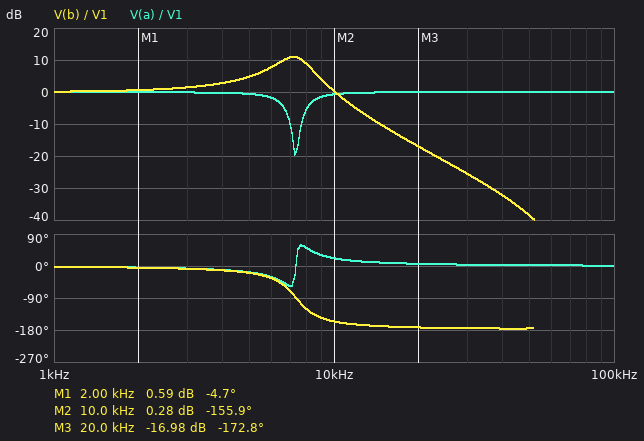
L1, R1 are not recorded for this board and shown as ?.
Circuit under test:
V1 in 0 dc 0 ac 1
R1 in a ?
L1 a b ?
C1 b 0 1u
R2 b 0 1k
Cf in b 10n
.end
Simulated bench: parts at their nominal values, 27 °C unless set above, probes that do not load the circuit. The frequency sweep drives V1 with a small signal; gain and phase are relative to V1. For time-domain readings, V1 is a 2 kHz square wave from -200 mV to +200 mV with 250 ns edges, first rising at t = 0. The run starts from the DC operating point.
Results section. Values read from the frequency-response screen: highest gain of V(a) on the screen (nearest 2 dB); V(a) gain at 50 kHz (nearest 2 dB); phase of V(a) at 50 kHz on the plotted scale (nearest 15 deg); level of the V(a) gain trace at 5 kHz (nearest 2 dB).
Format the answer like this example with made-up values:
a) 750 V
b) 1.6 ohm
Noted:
a) 0 dB
b) 0 dB
c) 0 deg
d) 0 dB
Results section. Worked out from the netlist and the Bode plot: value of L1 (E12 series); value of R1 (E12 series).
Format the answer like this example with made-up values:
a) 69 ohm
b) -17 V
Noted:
a) 470 µH
b) 5.6 Ω
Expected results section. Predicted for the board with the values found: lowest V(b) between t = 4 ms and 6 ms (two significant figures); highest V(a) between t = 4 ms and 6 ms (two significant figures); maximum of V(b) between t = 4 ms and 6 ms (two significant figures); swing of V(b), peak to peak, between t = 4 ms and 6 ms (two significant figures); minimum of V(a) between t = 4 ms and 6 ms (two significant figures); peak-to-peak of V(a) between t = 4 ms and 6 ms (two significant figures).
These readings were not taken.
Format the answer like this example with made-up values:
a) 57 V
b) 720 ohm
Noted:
a) -440 mV
b) 250 mV
c) 440 mV
d) 870 mV
e) -250 mV
f) 500 mV
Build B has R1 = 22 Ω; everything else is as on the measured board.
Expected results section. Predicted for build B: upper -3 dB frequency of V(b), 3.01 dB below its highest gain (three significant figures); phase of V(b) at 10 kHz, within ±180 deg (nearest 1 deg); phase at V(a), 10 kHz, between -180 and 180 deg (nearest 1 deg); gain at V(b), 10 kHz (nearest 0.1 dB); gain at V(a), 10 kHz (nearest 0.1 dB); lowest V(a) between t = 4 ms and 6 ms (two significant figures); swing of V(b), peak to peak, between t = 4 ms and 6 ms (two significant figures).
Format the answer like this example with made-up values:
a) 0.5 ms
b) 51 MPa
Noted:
a) 8.54 kHz
b) -120 deg
c) 56 deg
d) -4.6 dB
e) -5.6 dB
f) -230 mV
g) 510 mV
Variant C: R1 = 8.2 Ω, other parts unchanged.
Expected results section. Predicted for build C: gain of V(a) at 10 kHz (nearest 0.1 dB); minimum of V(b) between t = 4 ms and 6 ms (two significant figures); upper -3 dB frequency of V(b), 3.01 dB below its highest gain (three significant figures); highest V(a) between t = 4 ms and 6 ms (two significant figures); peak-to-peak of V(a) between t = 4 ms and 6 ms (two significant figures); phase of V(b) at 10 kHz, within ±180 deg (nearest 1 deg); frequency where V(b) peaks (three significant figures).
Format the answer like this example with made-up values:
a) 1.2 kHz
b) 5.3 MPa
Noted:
a) -1.4 dB
b) -400 mV
c) 8.39 kHz
d) 260 mV
e) 510 mV
f) -147 deg
g) 7.03 kHz
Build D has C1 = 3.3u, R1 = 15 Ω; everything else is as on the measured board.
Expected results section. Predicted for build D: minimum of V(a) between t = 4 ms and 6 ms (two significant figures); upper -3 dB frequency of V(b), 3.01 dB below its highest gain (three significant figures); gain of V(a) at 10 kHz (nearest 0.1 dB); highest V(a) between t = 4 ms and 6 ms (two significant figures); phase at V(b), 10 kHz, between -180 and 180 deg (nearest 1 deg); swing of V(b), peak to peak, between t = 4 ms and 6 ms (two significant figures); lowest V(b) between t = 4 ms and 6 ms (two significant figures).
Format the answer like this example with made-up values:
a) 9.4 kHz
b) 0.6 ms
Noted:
a) -220 mV
b) 4.41 kHz
c) -1.4 dB
d) 220 mV
e) -148 deg
f) 460 mV
g) -230 mV
